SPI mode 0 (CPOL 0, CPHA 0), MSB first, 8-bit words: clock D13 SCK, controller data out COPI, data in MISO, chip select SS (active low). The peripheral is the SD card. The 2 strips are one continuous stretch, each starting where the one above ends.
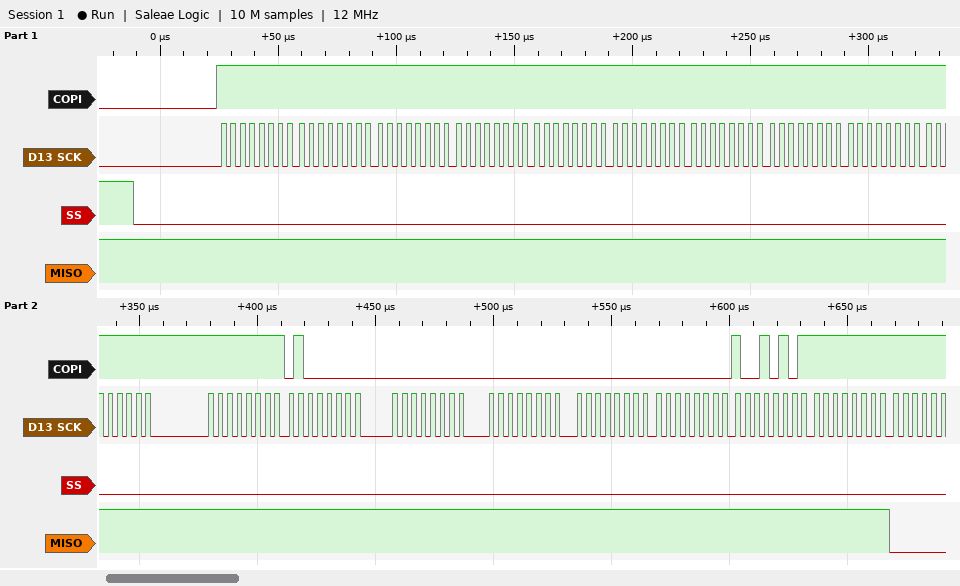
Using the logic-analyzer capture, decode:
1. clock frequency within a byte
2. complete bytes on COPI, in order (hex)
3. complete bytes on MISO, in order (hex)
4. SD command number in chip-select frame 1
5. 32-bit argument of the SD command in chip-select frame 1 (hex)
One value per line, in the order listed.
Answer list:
250 kHz
FF FF FF FF FF FF FF FF FF FF FF 40 00 00 00 00 95 FF
FF FF FF FF FF FF FF FF FF FF FF FF FF FF FF FF FF FF
CMD0
0x00000000
